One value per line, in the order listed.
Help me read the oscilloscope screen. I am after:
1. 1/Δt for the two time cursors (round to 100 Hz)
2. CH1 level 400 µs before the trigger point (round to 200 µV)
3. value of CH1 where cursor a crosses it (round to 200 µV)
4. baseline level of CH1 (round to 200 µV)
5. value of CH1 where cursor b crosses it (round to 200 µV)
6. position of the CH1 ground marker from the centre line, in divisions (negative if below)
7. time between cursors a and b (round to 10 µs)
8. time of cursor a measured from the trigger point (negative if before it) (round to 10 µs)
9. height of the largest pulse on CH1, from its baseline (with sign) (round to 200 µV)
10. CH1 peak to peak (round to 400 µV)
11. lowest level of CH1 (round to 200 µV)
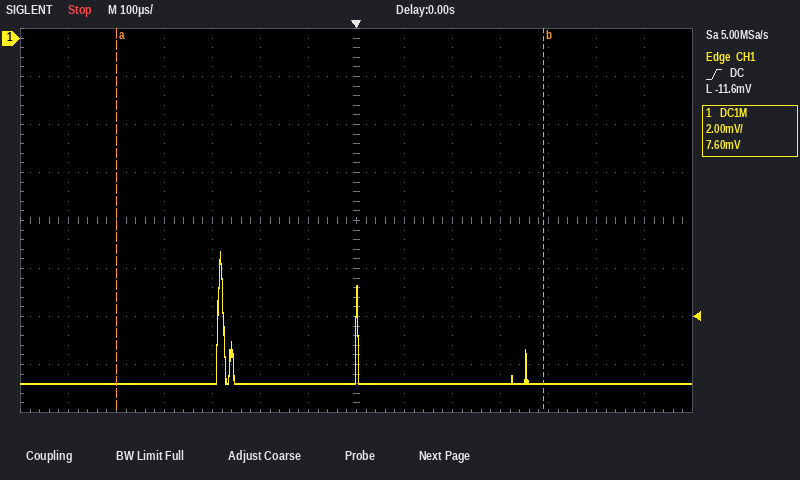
1.1 kHz
-14.4 mV
-14.4 mV
-14.4 mV
-14.4 mV
+3.8 div
890 µs
-500 µs
+5.4 mV
5.6 mV
-14.4 mV
